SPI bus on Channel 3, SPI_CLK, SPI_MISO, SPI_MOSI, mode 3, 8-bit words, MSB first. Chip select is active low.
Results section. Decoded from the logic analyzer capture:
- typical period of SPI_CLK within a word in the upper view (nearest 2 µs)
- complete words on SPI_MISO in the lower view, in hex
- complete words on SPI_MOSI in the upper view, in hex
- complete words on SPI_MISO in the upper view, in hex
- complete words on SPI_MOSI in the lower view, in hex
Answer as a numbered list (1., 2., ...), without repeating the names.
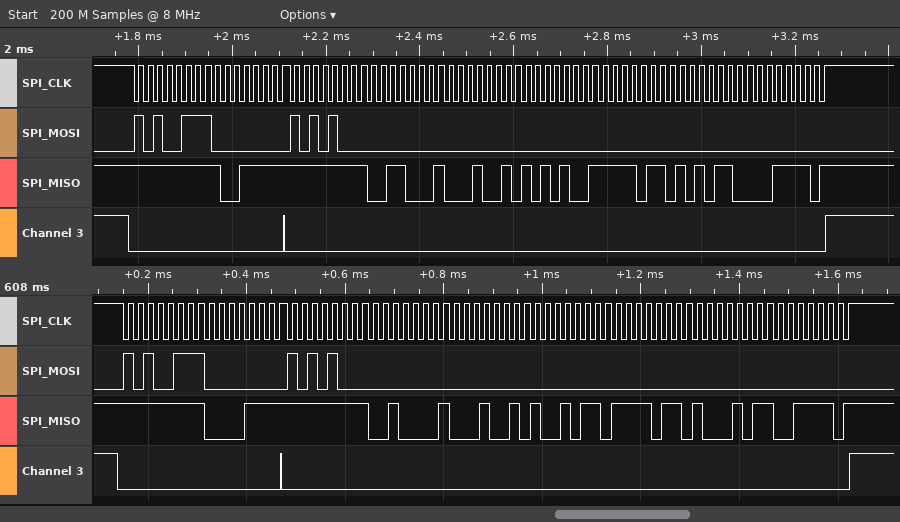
1. 20 µs
2. FF, 0F, FF, 21, 12, 96, F6, 8B, 3D
3. A7, 00, A8, 00, 00, 00, 00, 00, 00
4. FF, 9F, FF, 31, 12, A9, F6, AC, 3D
5. A7, 00, A8, 00, 00, 00, 00, 00, 00
